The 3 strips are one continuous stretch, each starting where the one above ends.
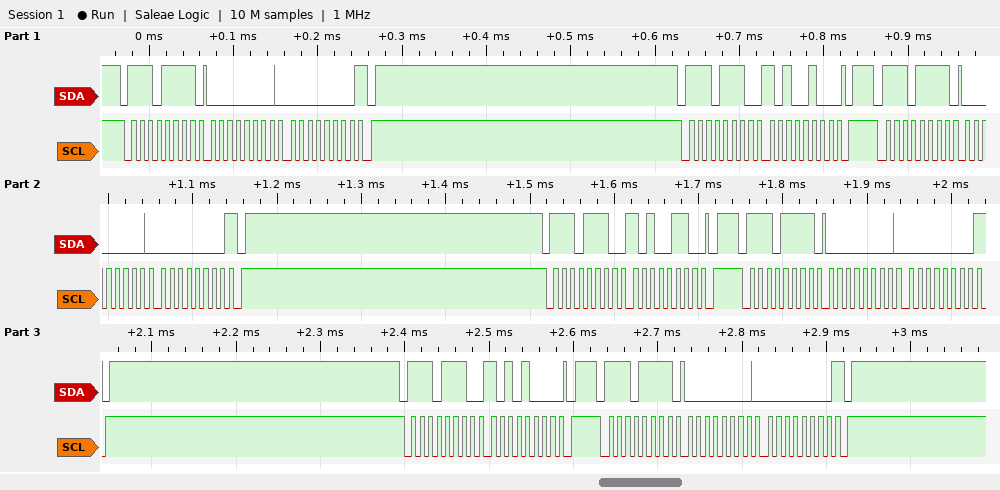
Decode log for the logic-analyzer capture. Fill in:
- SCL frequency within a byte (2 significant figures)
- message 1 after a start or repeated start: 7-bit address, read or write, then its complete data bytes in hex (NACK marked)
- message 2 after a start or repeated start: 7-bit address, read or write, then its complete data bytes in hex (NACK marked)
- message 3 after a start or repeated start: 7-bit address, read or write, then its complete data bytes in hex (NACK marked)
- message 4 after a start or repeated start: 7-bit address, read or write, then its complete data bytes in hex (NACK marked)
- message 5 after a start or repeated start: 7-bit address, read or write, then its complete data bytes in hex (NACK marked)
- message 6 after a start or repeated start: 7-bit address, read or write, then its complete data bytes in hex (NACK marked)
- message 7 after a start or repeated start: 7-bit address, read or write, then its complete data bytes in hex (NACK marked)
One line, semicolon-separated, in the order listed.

100 kHz; 0x77 read: 00 00 NACK; 0x77 write: A4; 0x77 read: 00 00 NACK; 0x77 write: A6; 0x77 read: 00 00 NACK; 0x77 write: A8; 0x77 read: 00 00 NACK
